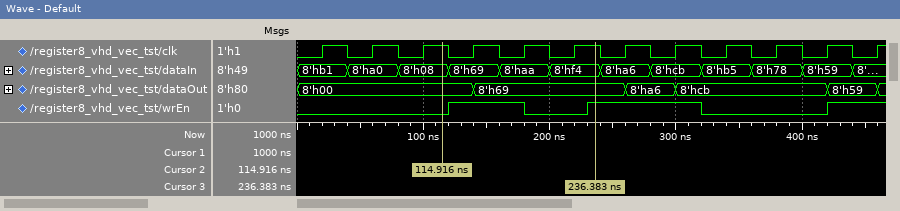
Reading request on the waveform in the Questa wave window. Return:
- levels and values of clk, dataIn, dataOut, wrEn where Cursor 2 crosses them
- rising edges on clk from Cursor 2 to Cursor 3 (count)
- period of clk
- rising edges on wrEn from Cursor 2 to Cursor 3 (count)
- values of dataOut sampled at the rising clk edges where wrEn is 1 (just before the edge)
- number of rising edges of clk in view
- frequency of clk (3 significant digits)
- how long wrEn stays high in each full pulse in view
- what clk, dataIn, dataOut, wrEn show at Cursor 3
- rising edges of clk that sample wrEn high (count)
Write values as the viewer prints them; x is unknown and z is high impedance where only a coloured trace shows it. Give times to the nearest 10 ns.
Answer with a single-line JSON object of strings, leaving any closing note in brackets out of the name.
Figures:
{"levels and values of clk, dataIn, dataOut, wrEn where Cursor 2 crosses them": "clk=1, dataIn=8'h08, dataOut=8'h00, wrEn=0", "rising edges on clk from Cursor 2 to Cursor 3": "3", "period of clk": "40 ns", "rising edges on wrEn from Cursor 2 to Cursor 3": "2", "values of dataOut sampled at the rising clk edges where wrEn is 1": "8'h00, 8'h69, 8'h69, 8'ha6, 8'h59", "number of rising edges of clk in view": "12", "frequency of clk": "25.0 MHz", "how long wrEn stays high in each full pulse in view": "60 ns, 90 ns", "what clk, dataIn, dataOut, wrEn show at Cursor 3": "clk=1, dataIn=8'hf4, dataOut=8'h69, wrEn=1", "rising edges of clk that sample wrEn high": "5"}
